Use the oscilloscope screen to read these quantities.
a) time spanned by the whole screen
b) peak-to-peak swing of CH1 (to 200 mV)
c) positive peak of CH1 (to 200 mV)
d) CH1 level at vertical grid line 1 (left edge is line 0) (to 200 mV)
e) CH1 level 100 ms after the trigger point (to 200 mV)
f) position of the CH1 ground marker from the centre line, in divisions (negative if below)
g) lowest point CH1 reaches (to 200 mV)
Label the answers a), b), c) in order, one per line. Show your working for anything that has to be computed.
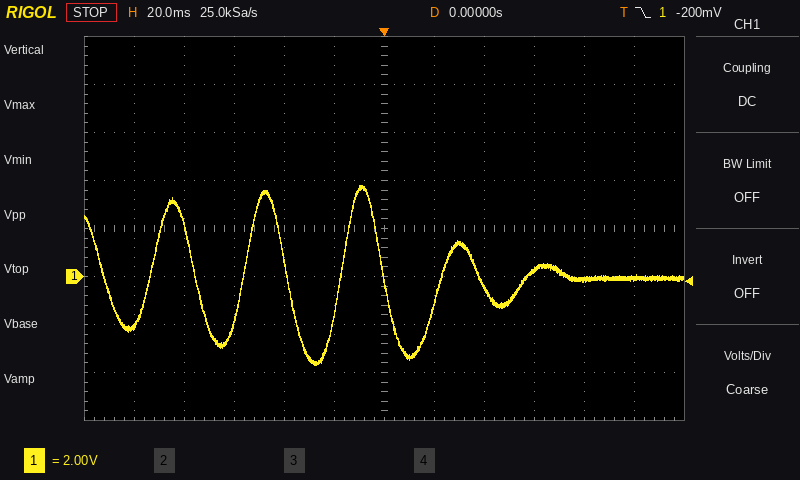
a) 240 ms
b) 3.8 V − (-3.6 V) = 7.4 V
c) 3.8 V
d) -2.0 V
e) 0.0 V
f) -1.0 div
g) -3.6 V
